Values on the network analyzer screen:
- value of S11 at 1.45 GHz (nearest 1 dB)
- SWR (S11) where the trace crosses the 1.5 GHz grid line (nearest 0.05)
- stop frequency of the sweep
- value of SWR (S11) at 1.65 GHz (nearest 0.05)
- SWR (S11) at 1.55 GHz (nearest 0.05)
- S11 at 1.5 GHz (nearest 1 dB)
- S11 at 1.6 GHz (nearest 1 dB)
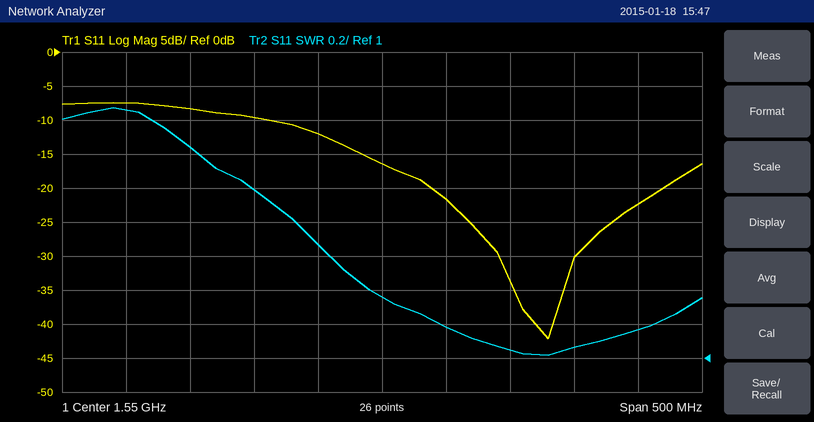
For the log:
-10 dB
1.65
1.8 GHz
1.05
1.35
-12 dB
-22 dB
